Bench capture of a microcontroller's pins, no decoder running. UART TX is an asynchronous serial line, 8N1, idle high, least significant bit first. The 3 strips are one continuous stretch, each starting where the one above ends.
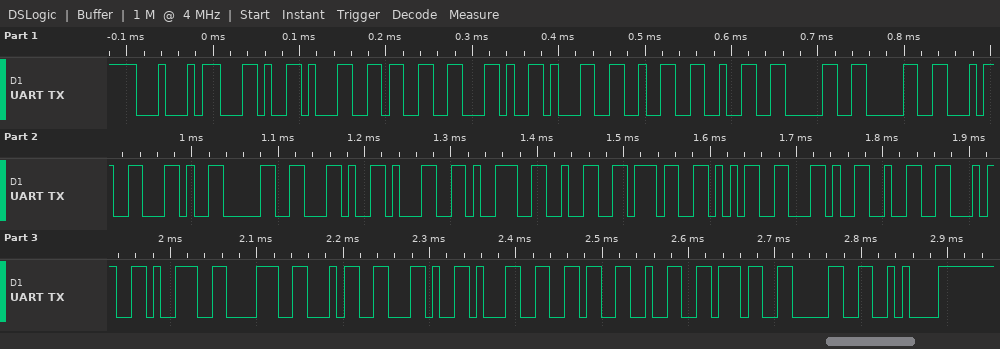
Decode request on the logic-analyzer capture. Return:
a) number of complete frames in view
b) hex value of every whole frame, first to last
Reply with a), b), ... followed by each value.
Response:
a) 32
b) 44 2C 31 33 2C 31 32 32 30 30 34 2C 30 2C 31 39 32 37 35 2C 32 34 39 38 34 2C 31 36 32 37 30 0A
